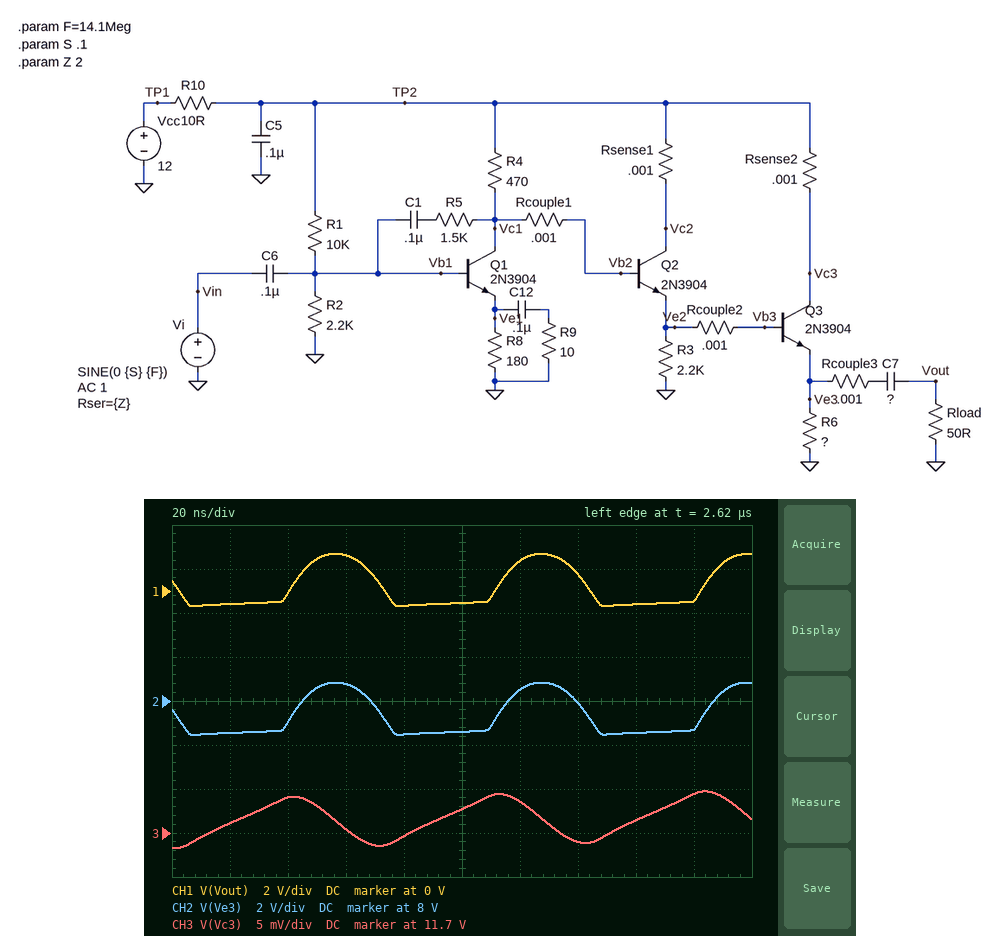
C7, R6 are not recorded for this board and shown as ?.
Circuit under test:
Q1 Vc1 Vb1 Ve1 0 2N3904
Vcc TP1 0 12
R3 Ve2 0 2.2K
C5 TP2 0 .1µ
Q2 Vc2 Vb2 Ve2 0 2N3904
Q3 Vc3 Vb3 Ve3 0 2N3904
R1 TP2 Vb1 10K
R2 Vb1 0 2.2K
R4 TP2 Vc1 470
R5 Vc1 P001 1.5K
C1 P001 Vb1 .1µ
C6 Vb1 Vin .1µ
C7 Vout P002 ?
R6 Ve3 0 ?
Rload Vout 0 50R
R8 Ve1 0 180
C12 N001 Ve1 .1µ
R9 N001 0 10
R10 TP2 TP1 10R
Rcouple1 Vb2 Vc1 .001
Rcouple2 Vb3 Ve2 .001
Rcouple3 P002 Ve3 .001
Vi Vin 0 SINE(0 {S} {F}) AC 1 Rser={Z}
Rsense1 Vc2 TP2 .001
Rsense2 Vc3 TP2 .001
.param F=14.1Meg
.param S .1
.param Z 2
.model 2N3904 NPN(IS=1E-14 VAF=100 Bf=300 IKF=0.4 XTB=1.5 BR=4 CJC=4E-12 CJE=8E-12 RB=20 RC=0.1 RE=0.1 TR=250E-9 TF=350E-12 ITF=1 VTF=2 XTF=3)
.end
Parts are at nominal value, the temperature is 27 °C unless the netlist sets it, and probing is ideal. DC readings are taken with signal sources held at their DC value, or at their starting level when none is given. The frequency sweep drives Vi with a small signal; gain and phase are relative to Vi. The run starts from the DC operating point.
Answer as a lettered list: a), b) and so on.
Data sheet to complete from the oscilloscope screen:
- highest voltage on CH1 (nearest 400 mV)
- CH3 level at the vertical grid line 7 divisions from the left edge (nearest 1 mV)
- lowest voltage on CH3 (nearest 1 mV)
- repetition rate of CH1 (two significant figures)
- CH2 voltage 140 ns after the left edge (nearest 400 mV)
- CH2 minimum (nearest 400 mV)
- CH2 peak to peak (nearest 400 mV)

a) 1.6 V
b) 11.694 V
c) 11.693 V
d) 14 MHz
e) 8.0 V
f) 6.4 V
g) 2.4 V
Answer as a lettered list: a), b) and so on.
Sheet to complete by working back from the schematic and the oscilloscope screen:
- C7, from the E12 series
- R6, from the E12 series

a) 47 nF
b) 560 Ω
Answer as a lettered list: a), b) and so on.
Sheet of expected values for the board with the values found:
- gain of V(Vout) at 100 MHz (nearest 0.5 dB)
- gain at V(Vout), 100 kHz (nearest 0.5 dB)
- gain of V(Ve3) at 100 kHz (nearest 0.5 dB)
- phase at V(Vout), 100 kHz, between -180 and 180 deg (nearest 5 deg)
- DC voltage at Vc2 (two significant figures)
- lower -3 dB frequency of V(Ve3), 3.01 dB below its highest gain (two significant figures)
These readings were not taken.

a) 20.0 dB
b) 21.0 dB
c) 22.5 dB
d) -95 deg
e) 12 V
f) 160 kHz
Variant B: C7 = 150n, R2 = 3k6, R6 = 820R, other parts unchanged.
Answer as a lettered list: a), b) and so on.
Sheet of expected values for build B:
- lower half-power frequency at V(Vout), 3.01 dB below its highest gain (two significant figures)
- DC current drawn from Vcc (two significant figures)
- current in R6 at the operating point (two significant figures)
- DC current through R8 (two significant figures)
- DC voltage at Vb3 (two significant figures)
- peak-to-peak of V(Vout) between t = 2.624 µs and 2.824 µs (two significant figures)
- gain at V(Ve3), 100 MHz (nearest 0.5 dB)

a) 180 kHz
b) 21 mA
c) 5.4 mA
d) 13 mA
e) 5.2 V
f) 2.6 V
g) 19.5 dB
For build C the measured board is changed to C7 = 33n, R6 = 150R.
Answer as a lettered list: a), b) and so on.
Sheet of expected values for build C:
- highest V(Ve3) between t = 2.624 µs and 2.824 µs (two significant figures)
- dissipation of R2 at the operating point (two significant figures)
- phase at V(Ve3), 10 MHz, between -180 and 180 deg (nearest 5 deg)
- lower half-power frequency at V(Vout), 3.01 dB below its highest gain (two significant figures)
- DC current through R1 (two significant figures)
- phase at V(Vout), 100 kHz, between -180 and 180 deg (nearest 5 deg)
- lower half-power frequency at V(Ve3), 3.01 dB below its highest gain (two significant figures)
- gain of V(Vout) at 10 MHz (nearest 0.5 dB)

a) 8.6 V
b) 1.9 mW
c) 165 deg
d) 210 kHz
e) 940 µA
f) -85 deg
g) 170 kHz
h) 28.0 dB
